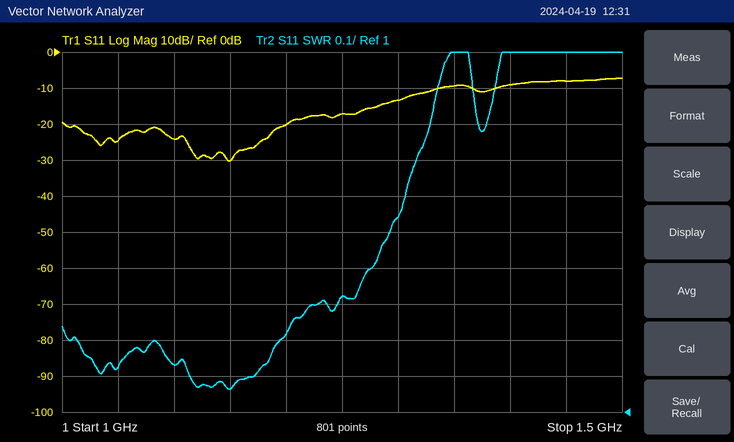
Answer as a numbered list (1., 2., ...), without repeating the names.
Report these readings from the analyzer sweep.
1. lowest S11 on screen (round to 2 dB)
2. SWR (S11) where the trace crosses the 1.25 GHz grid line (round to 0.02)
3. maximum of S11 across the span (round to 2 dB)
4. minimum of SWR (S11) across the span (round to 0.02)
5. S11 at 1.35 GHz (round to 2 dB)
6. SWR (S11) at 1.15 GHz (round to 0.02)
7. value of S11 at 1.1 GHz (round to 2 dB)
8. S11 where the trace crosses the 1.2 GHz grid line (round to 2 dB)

1. -30 dB
2. 1.32
3. -8 dB
4. 1.06
5. -10 dB
6. 1.06
7. -24 dB
8. -20 dB
